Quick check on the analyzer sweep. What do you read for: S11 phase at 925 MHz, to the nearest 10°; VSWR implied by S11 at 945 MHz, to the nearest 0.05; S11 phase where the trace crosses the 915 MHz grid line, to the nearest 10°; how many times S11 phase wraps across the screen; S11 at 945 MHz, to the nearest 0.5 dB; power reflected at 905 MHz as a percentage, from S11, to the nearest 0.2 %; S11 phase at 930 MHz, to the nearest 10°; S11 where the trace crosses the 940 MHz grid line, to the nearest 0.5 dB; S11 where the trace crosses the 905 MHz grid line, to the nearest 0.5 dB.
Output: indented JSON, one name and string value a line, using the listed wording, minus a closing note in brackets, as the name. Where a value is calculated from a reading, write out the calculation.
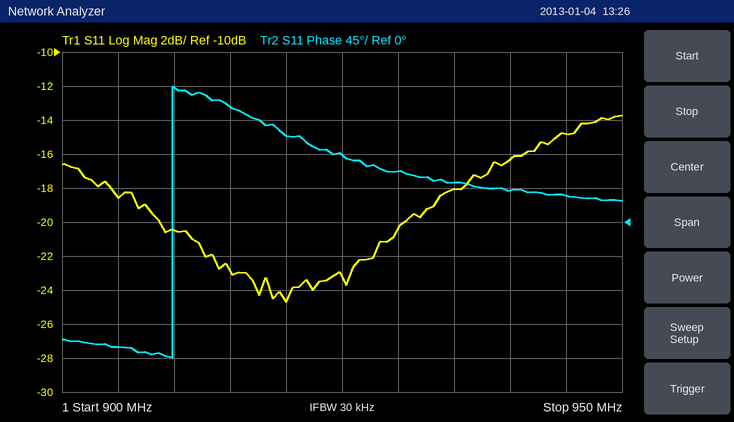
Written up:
{
  "S11 phase at 925 MHz, to the nearest 10°": "90°",
  "VSWR implied by S11 at 945 MHz, to the nearest 0.05": "|Γ| = 10^(-15/20) = 0.1778; VSWR = (1 + 0.1778)/(1 − 0.1778) ≈ 1.43, so 1.45 to the nearest 0.05",
  "S11 phase where the trace crosses the 915 MHz grid line, to the nearest 10°": "150°",
  "how many times S11 phase wraps across the screen": "1",
  "S11 at 945 MHz, to the nearest 0.5 dB": "-15.0 dB",
  "power reflected at 905 MHz as a percentage, from S11, to the nearest 0.2 %": "10^(-18.5/10) ≈ 1.4 %",
  "S11 phase at 930 MHz, to the nearest 10°": "70°",
  "S11 where the trace crosses the 940 MHz grid line, to the nearest 0.5 dB": "-16.5 dB",
  "S11 where the trace crosses the 905 MHz grid line, to the nearest 0.5 dB": "-18.5 dB"
}
